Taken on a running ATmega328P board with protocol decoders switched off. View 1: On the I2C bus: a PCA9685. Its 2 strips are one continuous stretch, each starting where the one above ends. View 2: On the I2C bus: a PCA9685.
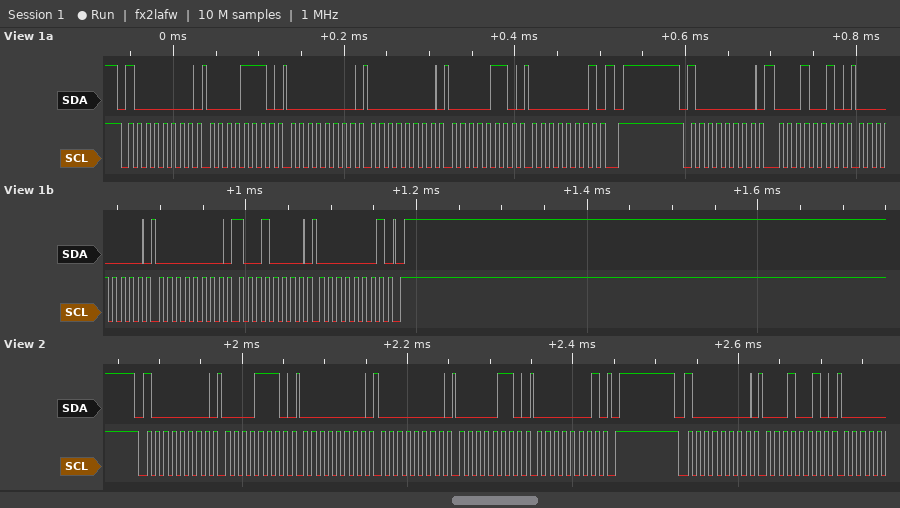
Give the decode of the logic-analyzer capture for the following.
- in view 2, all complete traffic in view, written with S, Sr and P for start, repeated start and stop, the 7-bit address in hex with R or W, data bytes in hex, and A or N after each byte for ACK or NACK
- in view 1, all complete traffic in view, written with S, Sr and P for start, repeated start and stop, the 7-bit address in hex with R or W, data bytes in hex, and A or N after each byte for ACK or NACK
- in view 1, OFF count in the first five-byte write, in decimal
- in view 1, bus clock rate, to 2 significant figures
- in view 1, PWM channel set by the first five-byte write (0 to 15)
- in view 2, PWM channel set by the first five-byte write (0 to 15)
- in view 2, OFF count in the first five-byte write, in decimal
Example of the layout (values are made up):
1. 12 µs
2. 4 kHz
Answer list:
1. S 40W A 0E A 00 A 00 A 06 A 01 A P S 40W A 12 A
2. S 40W A 0E A 00 A 00 A 06 A 01 A P S 40W A 12 A 00 A 00 A 90 A 01 A P
3. 262
4. 100 kHz
5. 2
6. 2
7. 262
